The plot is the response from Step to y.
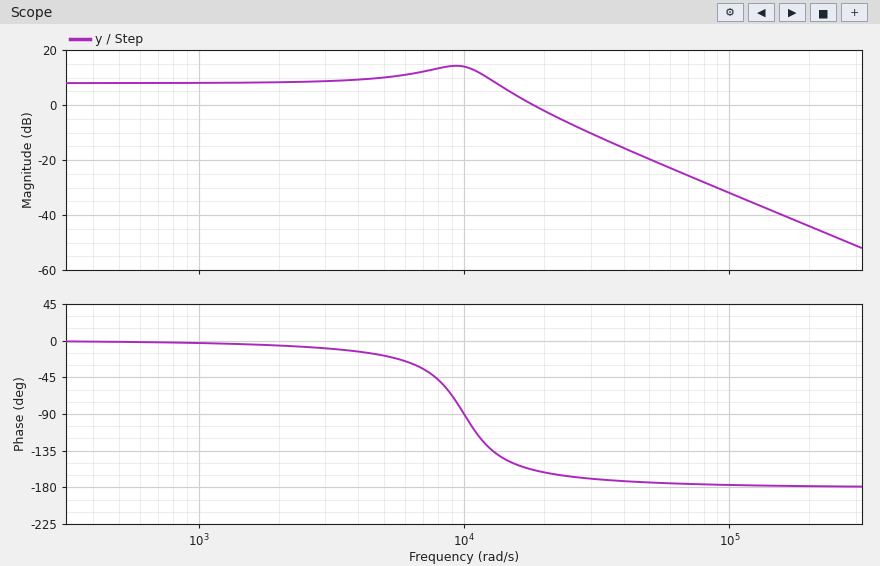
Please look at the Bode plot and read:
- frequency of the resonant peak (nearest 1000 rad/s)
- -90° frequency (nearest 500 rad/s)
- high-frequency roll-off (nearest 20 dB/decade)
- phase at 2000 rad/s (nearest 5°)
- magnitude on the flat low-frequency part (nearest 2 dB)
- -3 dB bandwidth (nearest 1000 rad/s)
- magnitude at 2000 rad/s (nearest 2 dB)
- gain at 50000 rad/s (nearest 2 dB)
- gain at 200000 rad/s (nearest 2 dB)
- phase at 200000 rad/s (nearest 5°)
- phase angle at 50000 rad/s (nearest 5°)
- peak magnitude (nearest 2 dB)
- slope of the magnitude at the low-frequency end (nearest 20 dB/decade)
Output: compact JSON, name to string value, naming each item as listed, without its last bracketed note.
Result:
{"frequency of the resonant peak": "9000 rad/s", "-90° frequency": "10000 rad/s", "high-frequency roll-off": "-40 dB/decade", "phase at 2000 rad/s": "-5°", "magnitude on the flat low-frequency part": "8 dB", "-3 dB bandwidth": "15000 rad/s", "magnitude at 2000 rad/s": "8 dB", "gain at 50000 rad/s": "-20 dB", "gain at 200000 rad/s": "-44 dB", "phase at 200000 rad/s": "-180°", "phase angle at 50000 rad/s": "-175°", "peak magnitude": "14 dB", "slope of the magnitude at the low-frequency end": "0 dB/decade"}
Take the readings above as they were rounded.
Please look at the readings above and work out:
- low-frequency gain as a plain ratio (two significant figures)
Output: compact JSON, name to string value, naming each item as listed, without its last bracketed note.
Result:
{"low-frequency gain as a plain ratio": "2.5"}
